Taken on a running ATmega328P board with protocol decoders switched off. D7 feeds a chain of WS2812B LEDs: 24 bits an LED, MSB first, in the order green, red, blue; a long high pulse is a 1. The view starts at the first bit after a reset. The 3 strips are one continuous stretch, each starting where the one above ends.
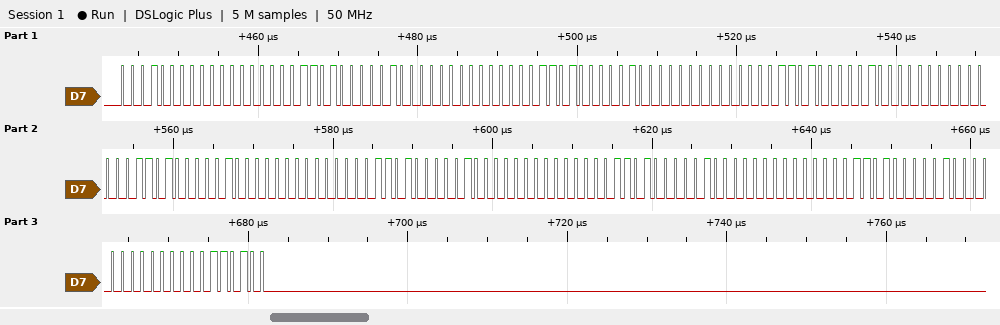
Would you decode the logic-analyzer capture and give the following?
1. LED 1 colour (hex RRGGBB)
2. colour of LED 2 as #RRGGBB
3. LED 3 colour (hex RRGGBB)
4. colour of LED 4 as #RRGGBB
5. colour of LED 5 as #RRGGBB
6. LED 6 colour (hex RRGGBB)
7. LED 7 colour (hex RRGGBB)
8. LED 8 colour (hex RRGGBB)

#001034
#001034
#001034
#001034
#001034
#001034
#001034
#001034
